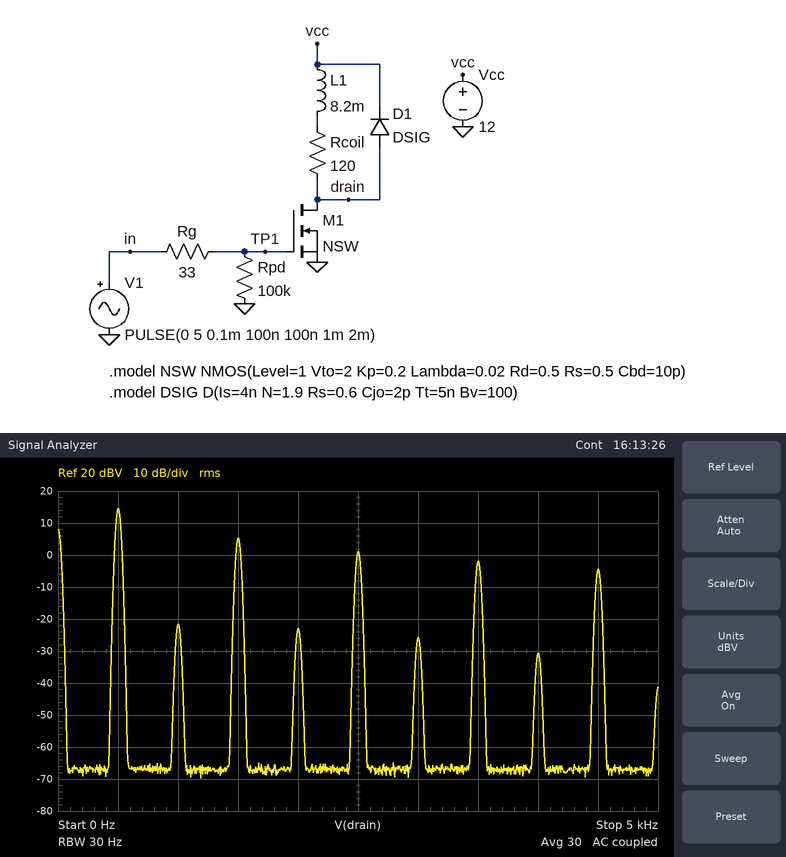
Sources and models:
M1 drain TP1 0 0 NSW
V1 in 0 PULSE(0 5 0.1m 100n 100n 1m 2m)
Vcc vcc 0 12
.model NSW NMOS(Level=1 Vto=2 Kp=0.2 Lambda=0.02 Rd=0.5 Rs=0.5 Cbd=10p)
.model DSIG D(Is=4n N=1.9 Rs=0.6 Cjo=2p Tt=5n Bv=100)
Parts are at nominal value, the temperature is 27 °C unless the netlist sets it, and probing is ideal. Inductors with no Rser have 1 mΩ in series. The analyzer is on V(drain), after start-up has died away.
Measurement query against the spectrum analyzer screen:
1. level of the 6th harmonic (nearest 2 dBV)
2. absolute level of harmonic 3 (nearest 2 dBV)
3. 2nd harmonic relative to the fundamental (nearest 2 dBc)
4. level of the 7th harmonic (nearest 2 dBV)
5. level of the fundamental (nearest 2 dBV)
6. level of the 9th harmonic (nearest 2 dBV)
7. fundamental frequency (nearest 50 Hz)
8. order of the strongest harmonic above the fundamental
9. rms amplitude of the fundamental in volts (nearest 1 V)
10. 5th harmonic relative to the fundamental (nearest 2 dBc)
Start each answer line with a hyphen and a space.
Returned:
- -26 dBV
- 6 dBV
- -36 dBc
- -2 dBV
- 14 dBV
- -4 dBV
- 500 Hz
- 3
- 5 V
- -14 dBc
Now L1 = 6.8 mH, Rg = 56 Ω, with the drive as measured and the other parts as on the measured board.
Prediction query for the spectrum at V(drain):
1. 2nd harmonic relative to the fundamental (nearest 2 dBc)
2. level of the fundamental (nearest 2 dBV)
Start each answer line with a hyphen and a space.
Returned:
- -38 dBc
- 14 dBV
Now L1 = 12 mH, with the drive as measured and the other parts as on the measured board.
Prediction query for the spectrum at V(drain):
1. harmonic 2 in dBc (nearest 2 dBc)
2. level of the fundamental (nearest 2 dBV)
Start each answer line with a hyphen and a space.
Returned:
- -34 dBc
- 14 dBV
